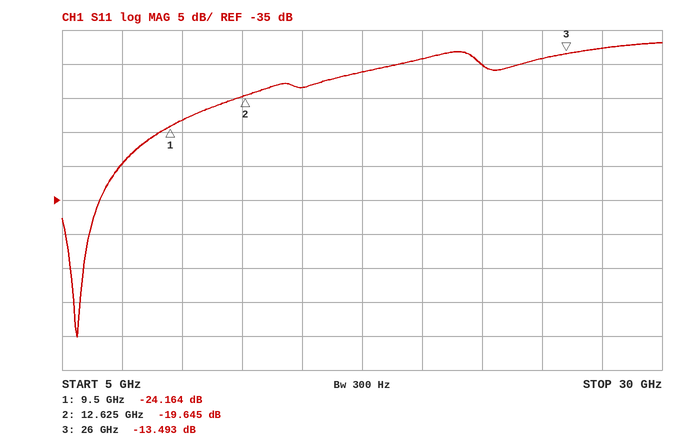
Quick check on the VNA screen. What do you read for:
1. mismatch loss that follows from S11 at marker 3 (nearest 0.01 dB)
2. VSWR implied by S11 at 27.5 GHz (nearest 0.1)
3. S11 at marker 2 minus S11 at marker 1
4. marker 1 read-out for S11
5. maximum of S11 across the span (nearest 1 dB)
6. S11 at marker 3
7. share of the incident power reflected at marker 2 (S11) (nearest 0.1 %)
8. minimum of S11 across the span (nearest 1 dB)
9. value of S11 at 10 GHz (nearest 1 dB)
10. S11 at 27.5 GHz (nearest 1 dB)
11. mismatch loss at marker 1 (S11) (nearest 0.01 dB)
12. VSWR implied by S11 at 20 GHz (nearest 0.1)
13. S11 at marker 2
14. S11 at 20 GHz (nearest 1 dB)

0.20 dB
1.6
4.519 dB
-24.164 dB
-12 dB
-13.493 dB
1.1 %
-55 dB
-23 dB
-13 dB
0.02 dB
1.5
-19.645 dB
-14 dB
